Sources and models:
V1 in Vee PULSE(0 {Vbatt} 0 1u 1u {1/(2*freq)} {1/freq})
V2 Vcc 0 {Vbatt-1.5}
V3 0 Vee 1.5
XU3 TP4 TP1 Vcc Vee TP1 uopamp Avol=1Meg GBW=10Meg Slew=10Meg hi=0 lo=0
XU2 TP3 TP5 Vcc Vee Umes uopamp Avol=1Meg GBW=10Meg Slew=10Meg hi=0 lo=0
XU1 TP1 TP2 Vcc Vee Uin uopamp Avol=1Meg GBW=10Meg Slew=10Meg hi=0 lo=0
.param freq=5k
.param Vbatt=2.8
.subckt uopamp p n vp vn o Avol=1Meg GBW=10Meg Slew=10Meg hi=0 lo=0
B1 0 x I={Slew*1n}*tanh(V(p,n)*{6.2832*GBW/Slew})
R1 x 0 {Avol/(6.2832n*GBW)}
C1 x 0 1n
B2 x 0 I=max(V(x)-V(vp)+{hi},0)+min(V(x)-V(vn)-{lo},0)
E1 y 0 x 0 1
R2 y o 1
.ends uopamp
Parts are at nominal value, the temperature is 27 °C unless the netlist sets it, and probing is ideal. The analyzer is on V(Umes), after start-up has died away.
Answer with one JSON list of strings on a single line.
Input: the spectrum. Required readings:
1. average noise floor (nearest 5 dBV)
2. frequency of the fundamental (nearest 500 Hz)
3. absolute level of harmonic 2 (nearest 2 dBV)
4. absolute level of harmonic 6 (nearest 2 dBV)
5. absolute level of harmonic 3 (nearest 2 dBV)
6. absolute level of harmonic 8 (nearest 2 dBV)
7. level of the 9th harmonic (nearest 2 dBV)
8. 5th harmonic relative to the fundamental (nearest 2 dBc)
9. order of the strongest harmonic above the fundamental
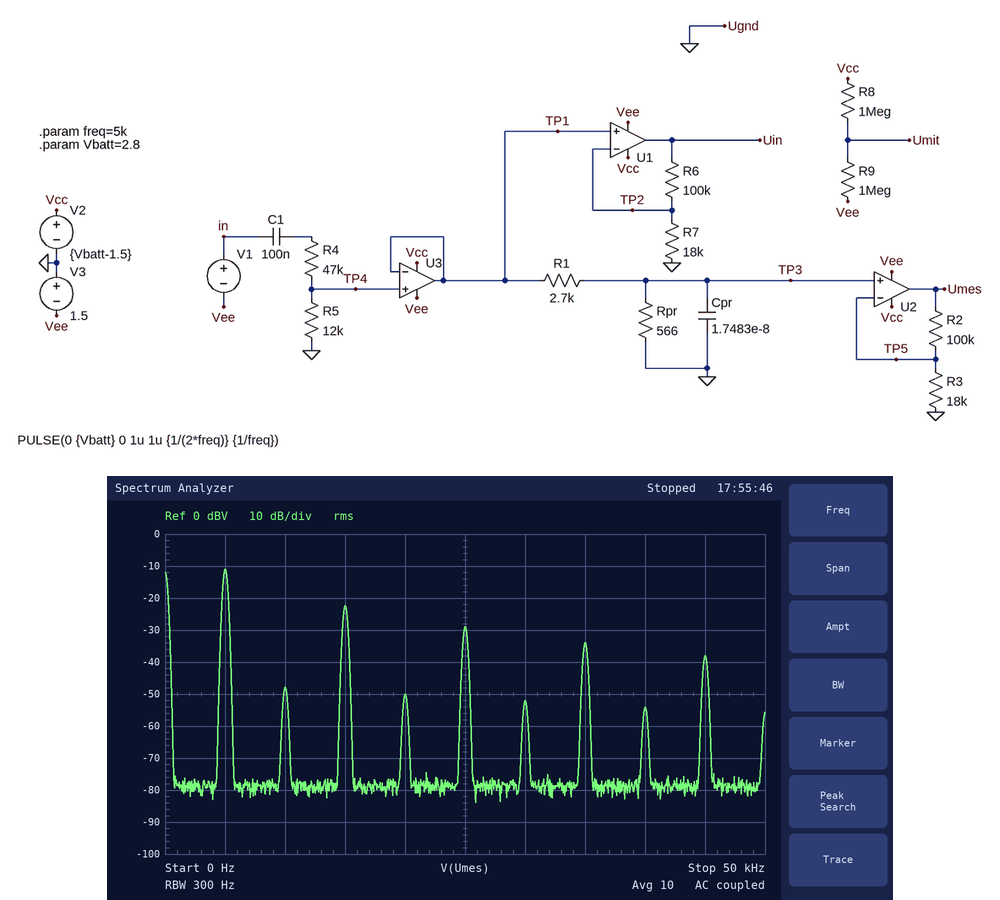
["-80 dBV", "5.0 kHz", "-48 dBV", "-52 dBV", "-22 dBV", "-54 dBV", "-38 dBV", "-18 dBc", "3"]
